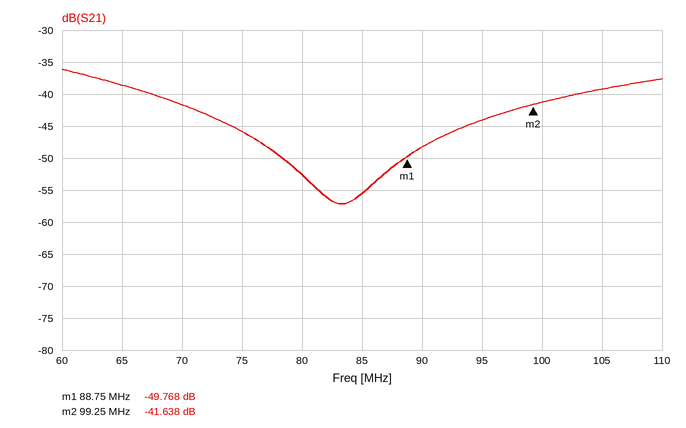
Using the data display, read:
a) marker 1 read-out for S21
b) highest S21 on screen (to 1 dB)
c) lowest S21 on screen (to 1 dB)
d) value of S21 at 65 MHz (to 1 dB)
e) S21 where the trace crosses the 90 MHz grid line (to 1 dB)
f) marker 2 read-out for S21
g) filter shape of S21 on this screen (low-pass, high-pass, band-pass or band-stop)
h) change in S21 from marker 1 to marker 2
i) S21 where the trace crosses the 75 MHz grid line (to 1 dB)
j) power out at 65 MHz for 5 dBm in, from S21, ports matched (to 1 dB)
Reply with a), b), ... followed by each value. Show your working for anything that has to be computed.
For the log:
a) -49.768 dB
b) -36 dB
c) -57 dB
d) -39 dB
e) -48 dB
f) -41.638 dB
g) band-stop
h) -41.638 − (-49.768) = 8.130 dB
i) -46 dB
j) 5 dBm + (-39 dB) = -34 dBm
